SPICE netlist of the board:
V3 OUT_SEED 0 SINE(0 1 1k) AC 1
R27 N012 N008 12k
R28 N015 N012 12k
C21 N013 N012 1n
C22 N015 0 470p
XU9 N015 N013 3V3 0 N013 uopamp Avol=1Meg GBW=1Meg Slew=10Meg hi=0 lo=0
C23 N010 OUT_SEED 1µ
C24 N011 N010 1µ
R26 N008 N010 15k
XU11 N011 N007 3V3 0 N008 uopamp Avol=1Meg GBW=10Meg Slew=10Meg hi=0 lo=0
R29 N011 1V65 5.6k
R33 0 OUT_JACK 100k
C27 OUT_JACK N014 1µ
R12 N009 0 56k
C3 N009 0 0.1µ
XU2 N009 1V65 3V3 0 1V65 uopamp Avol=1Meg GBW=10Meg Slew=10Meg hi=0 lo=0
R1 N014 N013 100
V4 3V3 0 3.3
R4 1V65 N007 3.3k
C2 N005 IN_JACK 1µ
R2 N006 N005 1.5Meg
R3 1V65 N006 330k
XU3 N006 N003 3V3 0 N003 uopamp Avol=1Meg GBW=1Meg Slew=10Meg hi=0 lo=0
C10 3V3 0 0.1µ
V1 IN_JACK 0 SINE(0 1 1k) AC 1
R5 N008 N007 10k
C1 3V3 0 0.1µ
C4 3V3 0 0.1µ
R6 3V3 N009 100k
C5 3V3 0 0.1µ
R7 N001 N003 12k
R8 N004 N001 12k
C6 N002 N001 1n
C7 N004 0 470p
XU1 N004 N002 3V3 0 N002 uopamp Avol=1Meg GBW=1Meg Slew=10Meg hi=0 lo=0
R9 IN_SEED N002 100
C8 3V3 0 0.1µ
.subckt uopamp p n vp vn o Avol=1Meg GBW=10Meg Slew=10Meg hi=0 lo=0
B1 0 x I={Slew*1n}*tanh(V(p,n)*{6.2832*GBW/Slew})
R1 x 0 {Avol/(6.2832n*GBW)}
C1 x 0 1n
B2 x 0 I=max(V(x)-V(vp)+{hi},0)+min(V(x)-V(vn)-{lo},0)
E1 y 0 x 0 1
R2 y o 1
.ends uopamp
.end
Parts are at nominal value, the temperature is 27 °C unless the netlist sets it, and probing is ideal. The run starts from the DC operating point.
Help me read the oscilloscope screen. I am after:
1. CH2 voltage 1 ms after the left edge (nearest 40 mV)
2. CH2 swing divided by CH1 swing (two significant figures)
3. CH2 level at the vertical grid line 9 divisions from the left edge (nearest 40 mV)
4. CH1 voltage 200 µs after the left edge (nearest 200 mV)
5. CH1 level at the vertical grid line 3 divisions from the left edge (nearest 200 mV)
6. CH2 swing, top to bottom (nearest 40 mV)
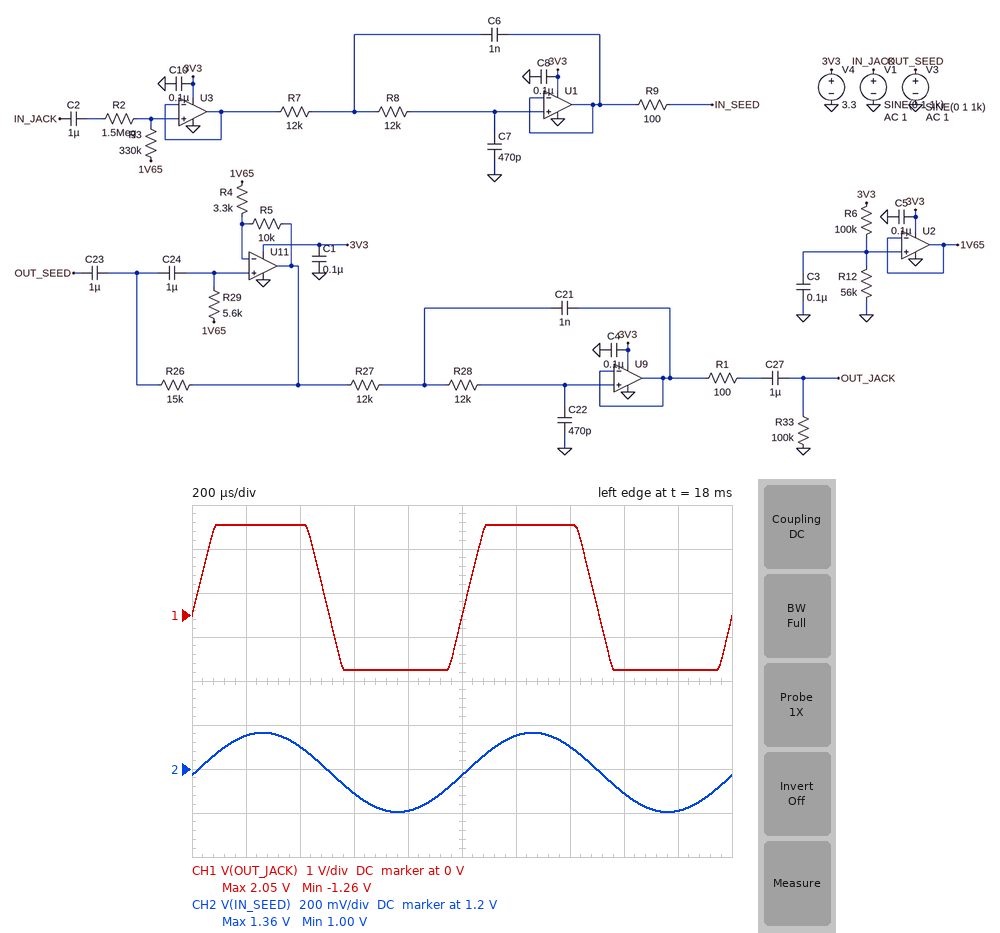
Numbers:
1.16 V
0.11
1.00 V
2.0 V
-1.2 V
360 mV
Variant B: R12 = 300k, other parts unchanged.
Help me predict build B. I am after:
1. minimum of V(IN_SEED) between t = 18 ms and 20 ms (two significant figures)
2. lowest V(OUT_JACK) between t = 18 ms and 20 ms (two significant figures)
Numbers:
2.3 V
-2.4 V
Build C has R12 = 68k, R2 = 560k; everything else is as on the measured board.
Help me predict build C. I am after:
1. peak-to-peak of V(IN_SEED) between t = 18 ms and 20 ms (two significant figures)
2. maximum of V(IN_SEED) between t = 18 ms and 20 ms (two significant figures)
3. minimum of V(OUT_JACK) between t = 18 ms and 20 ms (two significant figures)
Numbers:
740 mV
1.7 V
-1.4 V
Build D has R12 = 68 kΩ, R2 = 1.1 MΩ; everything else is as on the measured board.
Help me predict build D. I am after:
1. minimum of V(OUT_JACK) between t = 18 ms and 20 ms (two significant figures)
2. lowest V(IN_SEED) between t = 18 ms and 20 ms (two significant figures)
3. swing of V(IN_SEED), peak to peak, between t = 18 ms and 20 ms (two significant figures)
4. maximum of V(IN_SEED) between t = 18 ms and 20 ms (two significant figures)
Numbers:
-1.4 V
1.1 V
460 mV
1.6 V
